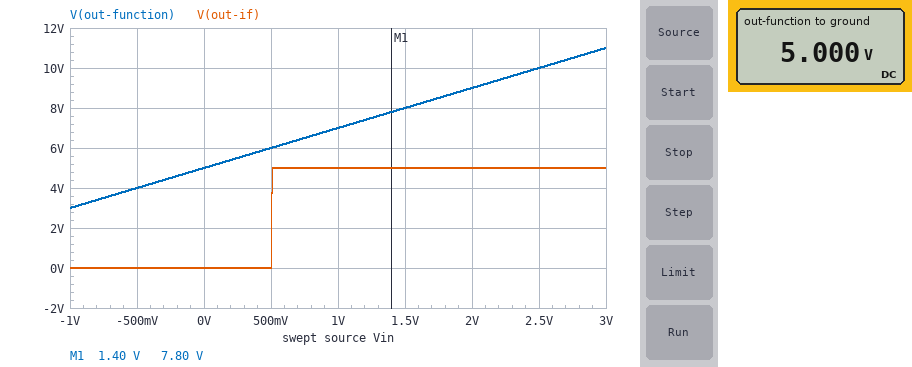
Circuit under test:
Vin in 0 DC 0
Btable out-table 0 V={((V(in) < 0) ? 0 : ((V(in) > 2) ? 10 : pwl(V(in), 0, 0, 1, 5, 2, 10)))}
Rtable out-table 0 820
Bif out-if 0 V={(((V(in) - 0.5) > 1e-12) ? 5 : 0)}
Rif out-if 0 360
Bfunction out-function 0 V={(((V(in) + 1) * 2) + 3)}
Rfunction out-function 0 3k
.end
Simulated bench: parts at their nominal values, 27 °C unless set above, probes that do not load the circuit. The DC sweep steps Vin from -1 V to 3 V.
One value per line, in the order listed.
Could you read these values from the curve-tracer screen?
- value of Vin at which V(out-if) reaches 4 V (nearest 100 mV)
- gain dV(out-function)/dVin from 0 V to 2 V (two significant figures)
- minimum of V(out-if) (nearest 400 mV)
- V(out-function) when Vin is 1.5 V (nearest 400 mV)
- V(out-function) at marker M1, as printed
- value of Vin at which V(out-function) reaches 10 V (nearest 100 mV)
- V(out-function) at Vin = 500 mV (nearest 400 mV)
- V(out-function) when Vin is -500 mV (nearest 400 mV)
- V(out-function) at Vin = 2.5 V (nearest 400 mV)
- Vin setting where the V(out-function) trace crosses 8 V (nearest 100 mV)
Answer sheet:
500 mV
2.0 V/V
0 V
8.0 V
7.80 V
2.5 V
6.0 V
4.0 V
10.0 V
1.5 V
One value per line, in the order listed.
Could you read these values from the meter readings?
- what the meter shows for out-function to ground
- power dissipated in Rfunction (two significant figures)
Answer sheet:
5.000 V
8.3 mW
